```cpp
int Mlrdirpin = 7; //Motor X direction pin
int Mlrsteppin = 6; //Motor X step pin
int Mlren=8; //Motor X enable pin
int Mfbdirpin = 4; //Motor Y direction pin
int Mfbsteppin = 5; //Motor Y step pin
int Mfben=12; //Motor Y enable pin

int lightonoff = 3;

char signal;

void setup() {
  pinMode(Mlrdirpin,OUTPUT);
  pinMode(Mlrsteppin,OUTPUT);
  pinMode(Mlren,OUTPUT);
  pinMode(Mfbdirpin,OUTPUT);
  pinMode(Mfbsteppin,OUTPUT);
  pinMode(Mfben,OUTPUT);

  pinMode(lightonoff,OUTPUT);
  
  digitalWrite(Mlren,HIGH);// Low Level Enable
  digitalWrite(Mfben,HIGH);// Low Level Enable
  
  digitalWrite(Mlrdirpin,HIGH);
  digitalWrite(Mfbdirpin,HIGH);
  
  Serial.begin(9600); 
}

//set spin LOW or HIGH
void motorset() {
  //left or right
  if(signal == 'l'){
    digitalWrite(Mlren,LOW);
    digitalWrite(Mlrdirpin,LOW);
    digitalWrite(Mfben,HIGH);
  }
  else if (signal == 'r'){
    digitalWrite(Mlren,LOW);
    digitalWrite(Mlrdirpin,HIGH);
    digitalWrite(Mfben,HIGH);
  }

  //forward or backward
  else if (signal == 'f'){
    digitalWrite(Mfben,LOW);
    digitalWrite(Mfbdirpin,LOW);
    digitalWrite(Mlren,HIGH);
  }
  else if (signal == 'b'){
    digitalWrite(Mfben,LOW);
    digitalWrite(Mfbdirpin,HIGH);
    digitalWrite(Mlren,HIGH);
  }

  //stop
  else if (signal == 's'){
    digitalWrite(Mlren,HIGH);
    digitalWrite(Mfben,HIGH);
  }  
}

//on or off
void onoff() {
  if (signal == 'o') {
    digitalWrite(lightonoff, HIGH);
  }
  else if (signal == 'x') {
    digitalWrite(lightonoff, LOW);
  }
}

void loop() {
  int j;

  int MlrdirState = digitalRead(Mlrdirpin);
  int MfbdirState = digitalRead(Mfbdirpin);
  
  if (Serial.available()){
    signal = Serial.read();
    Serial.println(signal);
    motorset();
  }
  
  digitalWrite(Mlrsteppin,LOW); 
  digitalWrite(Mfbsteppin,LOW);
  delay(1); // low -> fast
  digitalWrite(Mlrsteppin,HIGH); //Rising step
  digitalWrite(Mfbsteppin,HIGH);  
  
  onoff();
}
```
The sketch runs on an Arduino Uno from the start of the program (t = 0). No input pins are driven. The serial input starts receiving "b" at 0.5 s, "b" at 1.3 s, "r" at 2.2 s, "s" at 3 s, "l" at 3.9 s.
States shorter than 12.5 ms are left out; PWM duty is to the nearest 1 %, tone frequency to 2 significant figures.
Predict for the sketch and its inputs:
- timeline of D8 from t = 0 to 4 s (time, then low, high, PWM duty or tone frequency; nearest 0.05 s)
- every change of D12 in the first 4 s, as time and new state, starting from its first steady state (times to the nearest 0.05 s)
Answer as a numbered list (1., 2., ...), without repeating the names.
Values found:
1. 0 s high; 2.2 s low; 3 s high; 3.9 s low
2. 0 s high; 0.5 s low; 2.2 s high
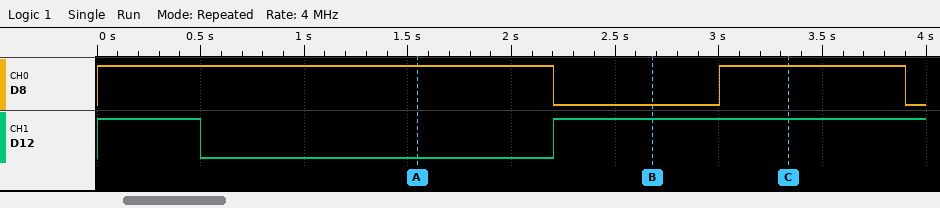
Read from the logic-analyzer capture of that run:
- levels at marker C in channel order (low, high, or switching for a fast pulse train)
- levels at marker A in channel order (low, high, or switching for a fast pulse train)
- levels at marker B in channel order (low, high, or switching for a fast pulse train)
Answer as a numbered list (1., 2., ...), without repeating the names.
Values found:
1. D8 high, D12 high
2. D8 high, D12 low
3. D8 low, D12 high
